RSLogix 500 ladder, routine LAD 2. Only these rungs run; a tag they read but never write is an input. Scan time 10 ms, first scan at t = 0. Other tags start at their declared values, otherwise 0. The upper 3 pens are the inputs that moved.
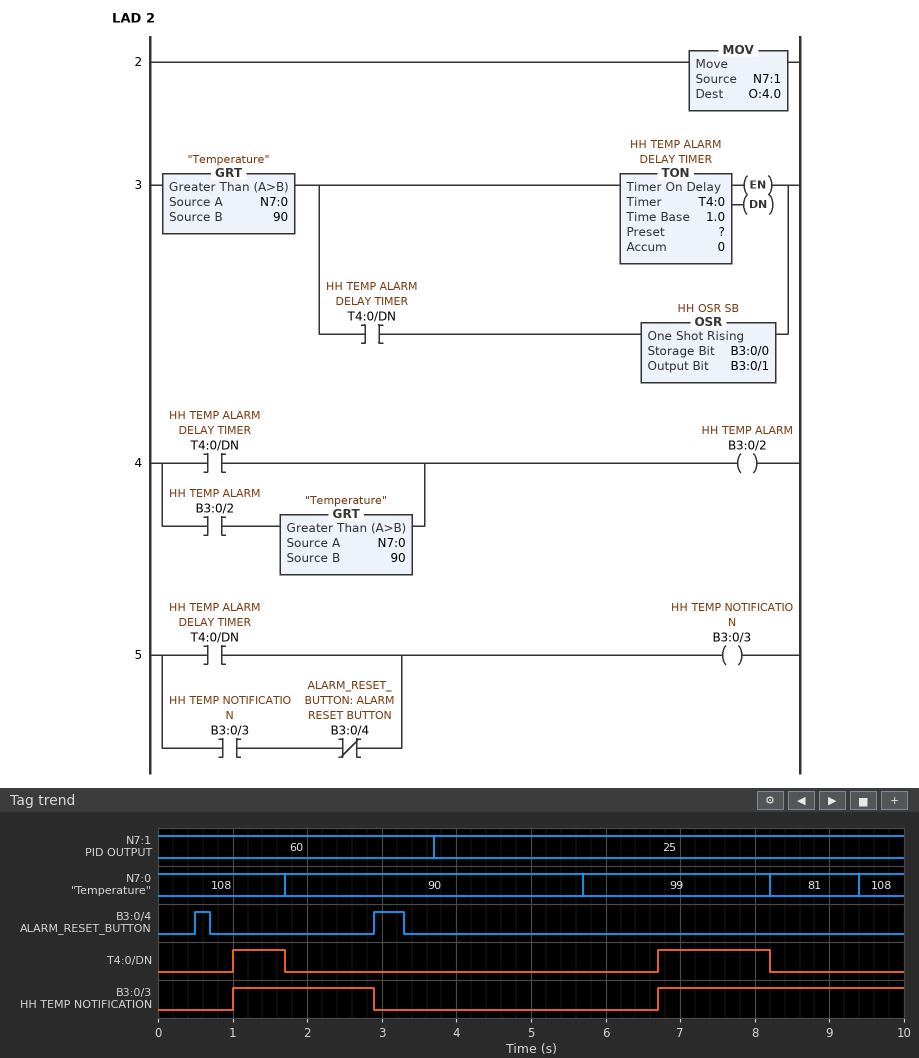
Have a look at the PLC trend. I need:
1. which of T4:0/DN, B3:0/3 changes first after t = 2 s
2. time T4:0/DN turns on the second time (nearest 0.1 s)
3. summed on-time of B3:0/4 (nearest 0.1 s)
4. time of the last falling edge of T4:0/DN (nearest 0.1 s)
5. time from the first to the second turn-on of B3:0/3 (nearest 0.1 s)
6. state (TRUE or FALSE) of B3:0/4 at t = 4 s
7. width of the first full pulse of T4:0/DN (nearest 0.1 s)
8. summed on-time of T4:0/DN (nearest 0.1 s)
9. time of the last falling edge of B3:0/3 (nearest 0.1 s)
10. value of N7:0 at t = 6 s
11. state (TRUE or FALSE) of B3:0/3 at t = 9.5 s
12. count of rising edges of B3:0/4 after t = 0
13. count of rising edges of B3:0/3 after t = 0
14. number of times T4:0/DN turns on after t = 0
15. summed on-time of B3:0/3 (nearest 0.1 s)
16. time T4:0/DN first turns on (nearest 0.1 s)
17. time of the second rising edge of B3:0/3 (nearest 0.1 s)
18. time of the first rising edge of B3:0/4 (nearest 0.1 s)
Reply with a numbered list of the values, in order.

1. B3:0/3
2. 6.7 s
3. 0.6 s
4. 8.2 s
5. 5.7 s
6. FALSE
7. 0.7 s
8. 2.2 s
9. 2.9 s
10. 99
11. TRUE
12. 2
13. 2
14. 2
15. 5.2 s
16. 1.0 s
17. 6.7 s
18. 0.5 s
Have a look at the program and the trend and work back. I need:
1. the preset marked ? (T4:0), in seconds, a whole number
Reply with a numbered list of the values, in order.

1. 1 s
